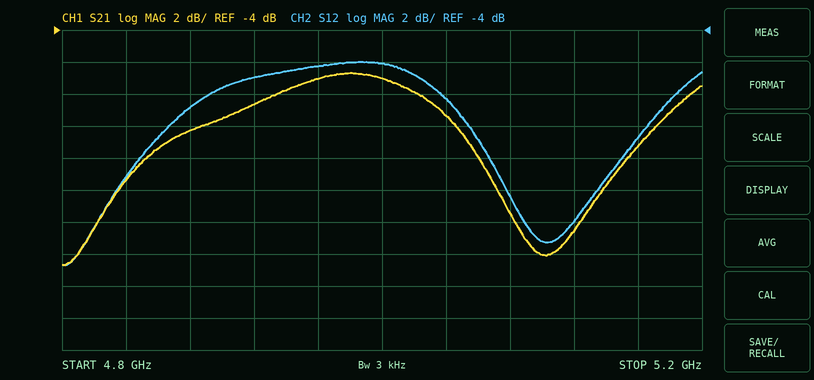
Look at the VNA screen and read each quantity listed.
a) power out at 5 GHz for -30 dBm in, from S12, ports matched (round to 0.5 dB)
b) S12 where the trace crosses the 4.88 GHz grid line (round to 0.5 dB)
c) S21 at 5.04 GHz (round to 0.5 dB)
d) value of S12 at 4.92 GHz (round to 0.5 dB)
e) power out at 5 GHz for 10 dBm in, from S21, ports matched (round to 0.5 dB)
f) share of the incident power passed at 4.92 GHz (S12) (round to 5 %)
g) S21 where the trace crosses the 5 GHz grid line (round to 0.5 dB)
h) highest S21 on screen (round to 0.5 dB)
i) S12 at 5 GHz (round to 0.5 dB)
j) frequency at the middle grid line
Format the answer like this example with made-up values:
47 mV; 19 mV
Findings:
-36.0 dBm; -9.0 dB; -9.5 dB; -7.0 dB; 3.0 dBm; 20 %; -7.0 dB; -6.5 dB; -6.0 dB; 5 GHz
